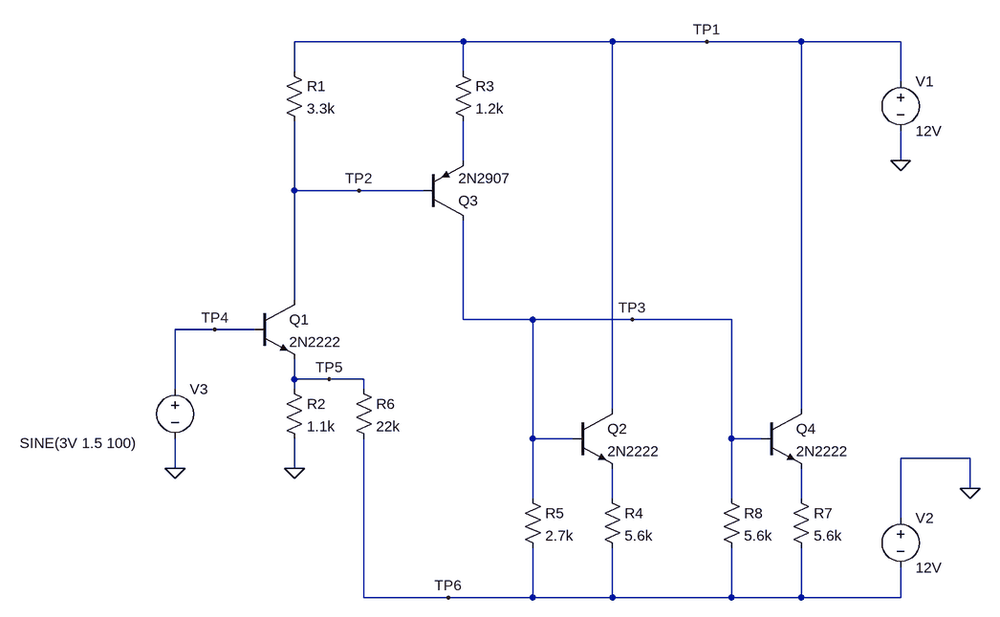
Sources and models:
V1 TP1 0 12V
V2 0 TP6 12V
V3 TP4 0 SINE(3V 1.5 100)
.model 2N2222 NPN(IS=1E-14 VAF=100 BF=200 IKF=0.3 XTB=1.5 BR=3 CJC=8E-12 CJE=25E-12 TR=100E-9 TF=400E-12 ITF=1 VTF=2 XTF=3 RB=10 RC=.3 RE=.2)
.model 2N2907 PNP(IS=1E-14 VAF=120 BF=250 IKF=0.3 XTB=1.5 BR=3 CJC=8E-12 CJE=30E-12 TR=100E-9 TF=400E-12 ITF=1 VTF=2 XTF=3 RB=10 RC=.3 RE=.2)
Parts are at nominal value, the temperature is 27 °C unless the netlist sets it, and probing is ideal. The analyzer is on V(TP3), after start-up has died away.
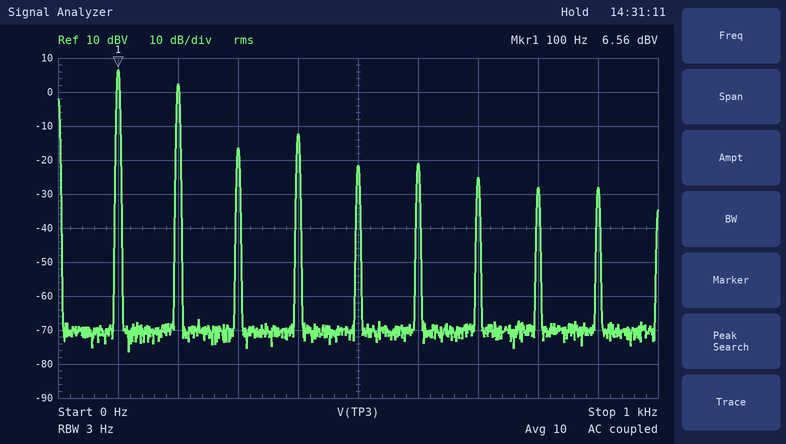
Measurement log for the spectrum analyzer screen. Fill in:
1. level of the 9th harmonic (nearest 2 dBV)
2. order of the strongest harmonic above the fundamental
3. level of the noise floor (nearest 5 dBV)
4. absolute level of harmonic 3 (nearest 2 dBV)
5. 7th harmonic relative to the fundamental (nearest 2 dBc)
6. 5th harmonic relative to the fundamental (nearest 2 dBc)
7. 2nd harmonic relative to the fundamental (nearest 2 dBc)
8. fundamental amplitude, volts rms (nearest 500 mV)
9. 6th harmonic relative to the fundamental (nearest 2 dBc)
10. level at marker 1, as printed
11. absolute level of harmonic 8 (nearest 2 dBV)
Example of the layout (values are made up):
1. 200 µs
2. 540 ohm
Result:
1. -28 dBV
2. 2
3. -70 dBV
4. -16 dBV
5. -32 dBc
6. -28 dBc
7. -4 dBc
8. 2.0 V
9. -28 dBc
10. 6.56 dBV
11. -28 dBV
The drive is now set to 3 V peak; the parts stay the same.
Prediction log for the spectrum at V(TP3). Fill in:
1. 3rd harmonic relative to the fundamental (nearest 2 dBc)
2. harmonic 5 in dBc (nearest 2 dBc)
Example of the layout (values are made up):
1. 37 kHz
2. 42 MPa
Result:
1. -22 dBc
2. -54 dBc
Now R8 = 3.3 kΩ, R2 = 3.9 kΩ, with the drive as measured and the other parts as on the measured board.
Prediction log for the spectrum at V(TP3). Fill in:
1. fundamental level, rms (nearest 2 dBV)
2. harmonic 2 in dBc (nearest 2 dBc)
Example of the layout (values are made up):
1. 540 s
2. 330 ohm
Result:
1. 2 dBV
2. -58 dBc
